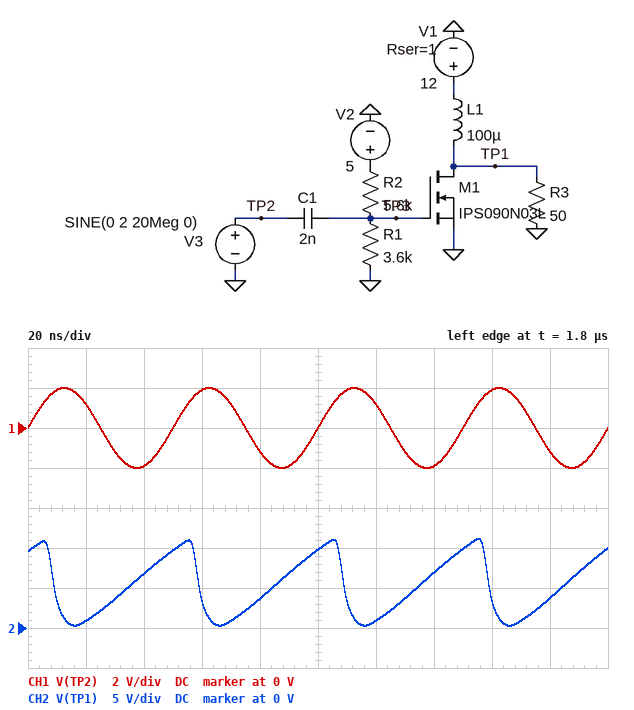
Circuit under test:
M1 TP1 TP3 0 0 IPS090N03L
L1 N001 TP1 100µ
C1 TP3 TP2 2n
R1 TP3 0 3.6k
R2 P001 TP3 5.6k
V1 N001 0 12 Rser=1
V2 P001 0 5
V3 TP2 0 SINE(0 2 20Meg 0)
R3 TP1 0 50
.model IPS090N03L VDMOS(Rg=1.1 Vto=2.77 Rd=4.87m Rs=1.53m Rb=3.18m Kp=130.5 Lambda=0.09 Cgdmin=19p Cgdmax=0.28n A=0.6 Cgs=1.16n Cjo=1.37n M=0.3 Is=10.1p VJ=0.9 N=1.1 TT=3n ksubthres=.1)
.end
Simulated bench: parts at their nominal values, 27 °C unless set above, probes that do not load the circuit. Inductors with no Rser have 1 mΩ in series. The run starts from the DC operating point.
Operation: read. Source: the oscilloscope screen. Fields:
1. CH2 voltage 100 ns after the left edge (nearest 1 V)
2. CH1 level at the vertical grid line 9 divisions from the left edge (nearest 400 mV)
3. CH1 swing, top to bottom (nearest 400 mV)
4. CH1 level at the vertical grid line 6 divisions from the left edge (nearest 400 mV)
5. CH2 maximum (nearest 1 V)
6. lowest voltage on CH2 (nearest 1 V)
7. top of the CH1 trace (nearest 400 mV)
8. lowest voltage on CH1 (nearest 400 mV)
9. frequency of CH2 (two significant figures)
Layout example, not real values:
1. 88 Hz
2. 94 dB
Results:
1. 10 V
2. -1.2 V
3. 4.0 V
4. 1.2 V
5. 11 V
6. 0 V
7. 2.0 V
8. -2.0 V
9. 20 MHz
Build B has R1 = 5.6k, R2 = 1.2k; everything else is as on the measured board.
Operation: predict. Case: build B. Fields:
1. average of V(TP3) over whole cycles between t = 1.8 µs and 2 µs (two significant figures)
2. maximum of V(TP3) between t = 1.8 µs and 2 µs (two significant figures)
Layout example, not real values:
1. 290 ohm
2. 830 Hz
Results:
1. 4.1 V
2. 5.3 V
